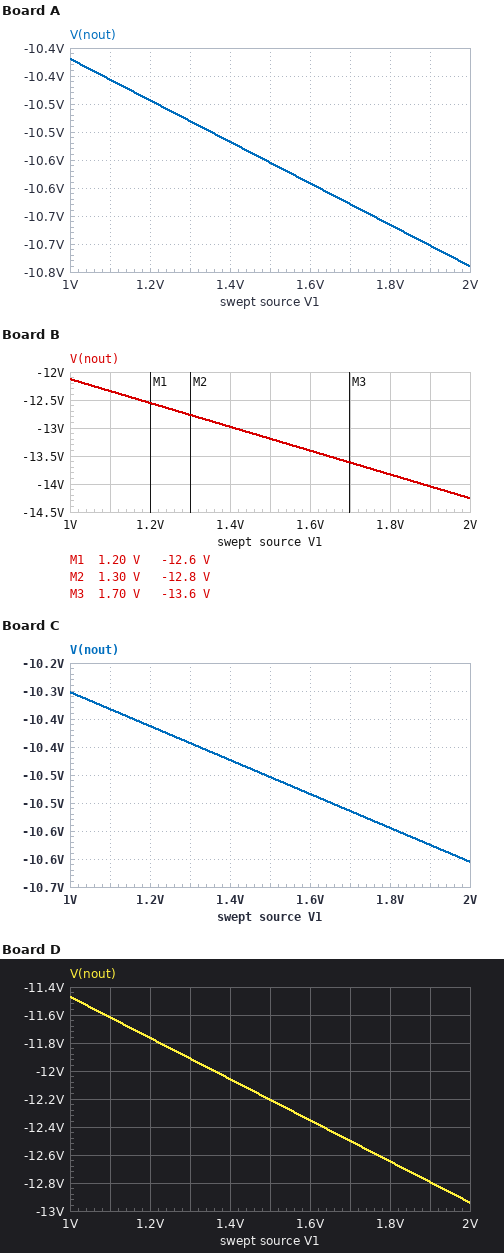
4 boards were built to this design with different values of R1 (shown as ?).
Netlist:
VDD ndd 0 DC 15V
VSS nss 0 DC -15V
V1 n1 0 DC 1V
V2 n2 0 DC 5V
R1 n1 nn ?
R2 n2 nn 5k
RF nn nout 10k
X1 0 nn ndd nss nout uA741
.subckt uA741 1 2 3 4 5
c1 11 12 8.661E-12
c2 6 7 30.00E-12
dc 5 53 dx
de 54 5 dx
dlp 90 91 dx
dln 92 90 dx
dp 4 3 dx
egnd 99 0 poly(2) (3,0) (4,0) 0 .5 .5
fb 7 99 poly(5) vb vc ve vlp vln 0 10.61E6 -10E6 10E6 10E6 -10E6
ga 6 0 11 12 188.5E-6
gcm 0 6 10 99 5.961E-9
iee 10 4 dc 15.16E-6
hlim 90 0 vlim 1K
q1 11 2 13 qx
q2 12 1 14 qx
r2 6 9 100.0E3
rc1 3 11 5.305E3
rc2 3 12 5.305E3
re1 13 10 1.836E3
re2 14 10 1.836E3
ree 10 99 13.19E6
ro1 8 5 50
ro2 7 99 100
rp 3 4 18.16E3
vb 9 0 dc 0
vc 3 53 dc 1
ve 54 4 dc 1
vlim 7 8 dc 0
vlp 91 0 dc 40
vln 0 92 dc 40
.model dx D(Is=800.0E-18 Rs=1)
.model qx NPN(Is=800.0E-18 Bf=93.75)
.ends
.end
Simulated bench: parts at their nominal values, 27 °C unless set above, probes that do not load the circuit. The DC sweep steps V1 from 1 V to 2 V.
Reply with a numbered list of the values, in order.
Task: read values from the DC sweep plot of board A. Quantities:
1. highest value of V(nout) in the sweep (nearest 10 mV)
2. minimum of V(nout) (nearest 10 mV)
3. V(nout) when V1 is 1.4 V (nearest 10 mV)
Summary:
1. -10.37 V
2. -10.74 V
3. -10.52 V
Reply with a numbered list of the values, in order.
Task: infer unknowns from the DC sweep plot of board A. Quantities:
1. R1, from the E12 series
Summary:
1. 27 kΩ
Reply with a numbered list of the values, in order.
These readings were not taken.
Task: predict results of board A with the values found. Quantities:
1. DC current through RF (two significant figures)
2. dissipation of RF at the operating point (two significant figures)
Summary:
1. 1.0 mA
2. 11 mW
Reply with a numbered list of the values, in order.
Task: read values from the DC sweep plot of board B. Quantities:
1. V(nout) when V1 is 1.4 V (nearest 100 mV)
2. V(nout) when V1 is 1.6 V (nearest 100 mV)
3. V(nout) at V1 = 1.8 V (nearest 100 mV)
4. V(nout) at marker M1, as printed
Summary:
1. -13.0 V
2. -13.4 V
3. -13.8 V
4. -12.6 V
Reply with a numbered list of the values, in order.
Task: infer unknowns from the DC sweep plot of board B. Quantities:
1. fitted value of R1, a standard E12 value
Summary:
1. 4.7 kΩ
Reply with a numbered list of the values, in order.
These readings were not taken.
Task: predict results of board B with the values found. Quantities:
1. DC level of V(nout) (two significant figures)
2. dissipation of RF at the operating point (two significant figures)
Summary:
1. -12 V
2. 15 mW
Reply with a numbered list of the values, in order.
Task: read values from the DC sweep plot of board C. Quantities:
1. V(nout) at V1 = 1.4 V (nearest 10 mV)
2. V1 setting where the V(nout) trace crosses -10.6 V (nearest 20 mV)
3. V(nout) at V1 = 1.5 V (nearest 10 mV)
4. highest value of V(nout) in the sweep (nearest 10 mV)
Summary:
1. -10.42 V
2. 1.82 V
3. -10.45 V
4. -10.30 V
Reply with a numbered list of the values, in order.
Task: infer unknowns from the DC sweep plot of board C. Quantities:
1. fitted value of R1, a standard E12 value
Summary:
1. 33 kΩ
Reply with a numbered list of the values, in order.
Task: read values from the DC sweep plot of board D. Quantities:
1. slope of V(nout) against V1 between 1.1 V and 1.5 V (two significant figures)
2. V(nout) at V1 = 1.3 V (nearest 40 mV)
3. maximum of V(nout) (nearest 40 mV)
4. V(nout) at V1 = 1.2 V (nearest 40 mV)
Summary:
1. -1.5 V/V
2. -11.92 V
3. -11.48 V
4. -11.76 V
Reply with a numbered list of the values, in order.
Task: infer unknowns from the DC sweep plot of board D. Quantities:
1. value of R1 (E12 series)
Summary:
1. 6.8 kΩ
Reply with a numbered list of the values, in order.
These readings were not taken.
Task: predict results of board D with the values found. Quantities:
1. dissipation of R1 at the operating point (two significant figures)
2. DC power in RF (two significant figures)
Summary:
1. 150 µW
2. 13 mW
